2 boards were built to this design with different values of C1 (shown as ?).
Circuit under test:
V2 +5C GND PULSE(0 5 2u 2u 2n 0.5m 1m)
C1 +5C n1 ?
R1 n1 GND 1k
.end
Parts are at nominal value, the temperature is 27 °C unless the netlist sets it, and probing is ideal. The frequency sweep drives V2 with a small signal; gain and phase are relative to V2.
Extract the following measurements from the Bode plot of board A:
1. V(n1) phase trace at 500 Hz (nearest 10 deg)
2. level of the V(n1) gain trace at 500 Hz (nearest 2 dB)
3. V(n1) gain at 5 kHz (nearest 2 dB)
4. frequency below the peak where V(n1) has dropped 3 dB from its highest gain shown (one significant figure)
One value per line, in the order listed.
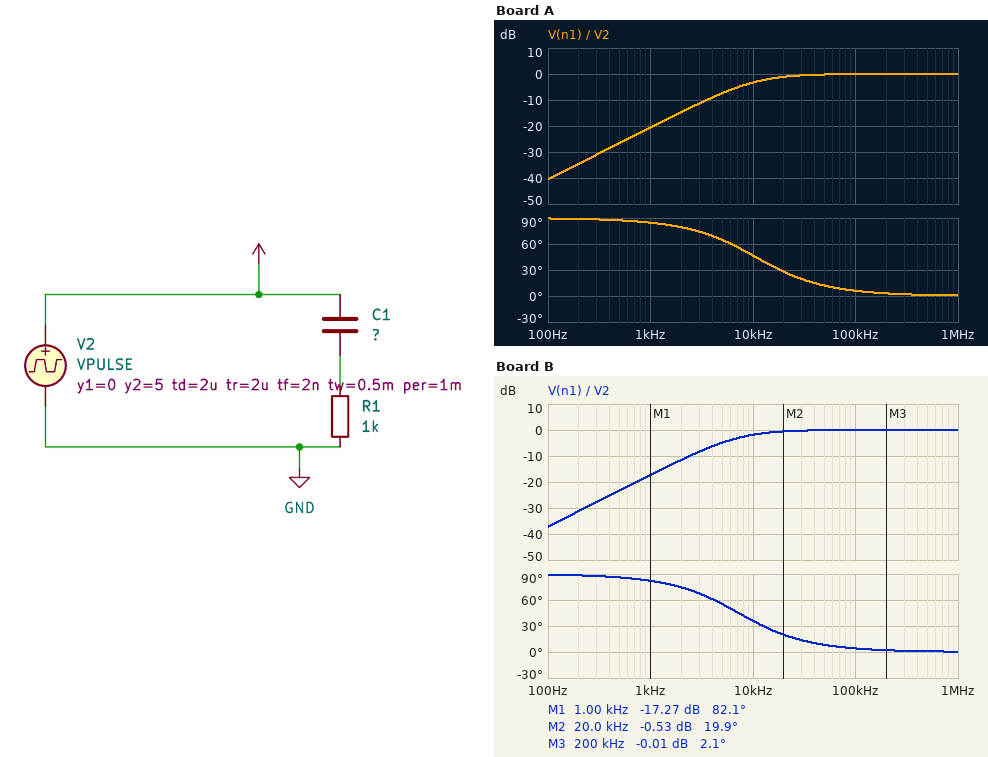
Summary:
90 deg
-26 dB
-8 dB
10 kHz
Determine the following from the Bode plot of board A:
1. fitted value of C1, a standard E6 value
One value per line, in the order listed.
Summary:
15 nF
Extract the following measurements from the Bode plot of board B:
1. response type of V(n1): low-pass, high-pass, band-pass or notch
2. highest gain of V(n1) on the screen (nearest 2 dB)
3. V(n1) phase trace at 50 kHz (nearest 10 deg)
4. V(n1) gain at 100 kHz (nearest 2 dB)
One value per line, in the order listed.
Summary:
high-pass
0 dB
10 deg
0 dB
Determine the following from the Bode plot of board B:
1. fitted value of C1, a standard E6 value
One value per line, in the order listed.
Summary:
22 nF
